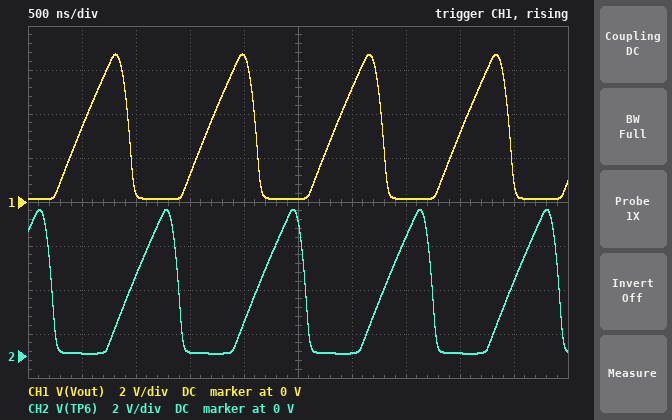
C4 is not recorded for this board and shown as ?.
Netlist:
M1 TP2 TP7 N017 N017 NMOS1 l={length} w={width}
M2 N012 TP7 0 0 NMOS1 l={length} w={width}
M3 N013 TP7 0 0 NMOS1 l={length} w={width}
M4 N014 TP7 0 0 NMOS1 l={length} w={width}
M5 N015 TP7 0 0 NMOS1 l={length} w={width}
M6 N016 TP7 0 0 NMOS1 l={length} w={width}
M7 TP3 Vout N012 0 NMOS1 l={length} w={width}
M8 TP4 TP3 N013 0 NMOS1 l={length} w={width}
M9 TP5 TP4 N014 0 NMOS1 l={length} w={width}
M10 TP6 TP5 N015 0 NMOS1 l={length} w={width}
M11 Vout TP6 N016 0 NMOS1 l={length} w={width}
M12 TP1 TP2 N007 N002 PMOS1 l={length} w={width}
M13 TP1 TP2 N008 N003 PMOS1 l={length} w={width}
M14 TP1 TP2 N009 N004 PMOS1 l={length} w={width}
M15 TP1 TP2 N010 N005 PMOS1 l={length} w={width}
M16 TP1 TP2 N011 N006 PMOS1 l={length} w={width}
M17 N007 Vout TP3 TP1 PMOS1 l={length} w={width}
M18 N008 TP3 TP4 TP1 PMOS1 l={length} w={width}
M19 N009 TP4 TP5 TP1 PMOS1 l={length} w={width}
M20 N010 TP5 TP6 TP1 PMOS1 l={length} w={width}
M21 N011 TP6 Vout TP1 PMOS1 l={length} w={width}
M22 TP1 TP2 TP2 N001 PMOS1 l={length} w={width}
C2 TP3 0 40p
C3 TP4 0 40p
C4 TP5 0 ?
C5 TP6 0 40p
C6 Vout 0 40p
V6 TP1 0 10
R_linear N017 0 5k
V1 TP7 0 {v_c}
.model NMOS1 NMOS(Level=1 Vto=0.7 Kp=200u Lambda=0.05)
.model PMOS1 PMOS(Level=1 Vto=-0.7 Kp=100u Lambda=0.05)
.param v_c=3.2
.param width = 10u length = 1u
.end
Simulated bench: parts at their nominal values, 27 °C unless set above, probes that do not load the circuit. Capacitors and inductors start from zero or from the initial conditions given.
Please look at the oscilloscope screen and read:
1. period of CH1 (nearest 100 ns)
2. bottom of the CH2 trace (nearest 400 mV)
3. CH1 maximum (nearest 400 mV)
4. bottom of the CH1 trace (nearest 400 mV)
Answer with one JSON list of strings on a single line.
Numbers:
["1.2 µs", "0 V", "6.8 V", "0 V"]
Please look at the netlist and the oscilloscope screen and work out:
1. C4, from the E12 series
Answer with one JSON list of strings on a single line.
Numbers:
["33 pF"]
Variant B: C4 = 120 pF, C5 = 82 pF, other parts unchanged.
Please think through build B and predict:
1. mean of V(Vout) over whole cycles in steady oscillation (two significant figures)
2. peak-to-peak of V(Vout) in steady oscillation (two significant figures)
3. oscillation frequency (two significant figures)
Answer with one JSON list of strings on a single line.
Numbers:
["2.7 V", "8.1 V", "530 kHz"]
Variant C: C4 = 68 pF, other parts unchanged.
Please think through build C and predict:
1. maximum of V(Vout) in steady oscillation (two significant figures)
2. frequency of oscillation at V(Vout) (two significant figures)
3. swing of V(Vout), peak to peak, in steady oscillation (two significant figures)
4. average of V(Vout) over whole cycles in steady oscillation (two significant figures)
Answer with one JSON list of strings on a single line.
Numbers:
["7.1 V", "730 kHz", "7.0 V", "2.4 V"]
